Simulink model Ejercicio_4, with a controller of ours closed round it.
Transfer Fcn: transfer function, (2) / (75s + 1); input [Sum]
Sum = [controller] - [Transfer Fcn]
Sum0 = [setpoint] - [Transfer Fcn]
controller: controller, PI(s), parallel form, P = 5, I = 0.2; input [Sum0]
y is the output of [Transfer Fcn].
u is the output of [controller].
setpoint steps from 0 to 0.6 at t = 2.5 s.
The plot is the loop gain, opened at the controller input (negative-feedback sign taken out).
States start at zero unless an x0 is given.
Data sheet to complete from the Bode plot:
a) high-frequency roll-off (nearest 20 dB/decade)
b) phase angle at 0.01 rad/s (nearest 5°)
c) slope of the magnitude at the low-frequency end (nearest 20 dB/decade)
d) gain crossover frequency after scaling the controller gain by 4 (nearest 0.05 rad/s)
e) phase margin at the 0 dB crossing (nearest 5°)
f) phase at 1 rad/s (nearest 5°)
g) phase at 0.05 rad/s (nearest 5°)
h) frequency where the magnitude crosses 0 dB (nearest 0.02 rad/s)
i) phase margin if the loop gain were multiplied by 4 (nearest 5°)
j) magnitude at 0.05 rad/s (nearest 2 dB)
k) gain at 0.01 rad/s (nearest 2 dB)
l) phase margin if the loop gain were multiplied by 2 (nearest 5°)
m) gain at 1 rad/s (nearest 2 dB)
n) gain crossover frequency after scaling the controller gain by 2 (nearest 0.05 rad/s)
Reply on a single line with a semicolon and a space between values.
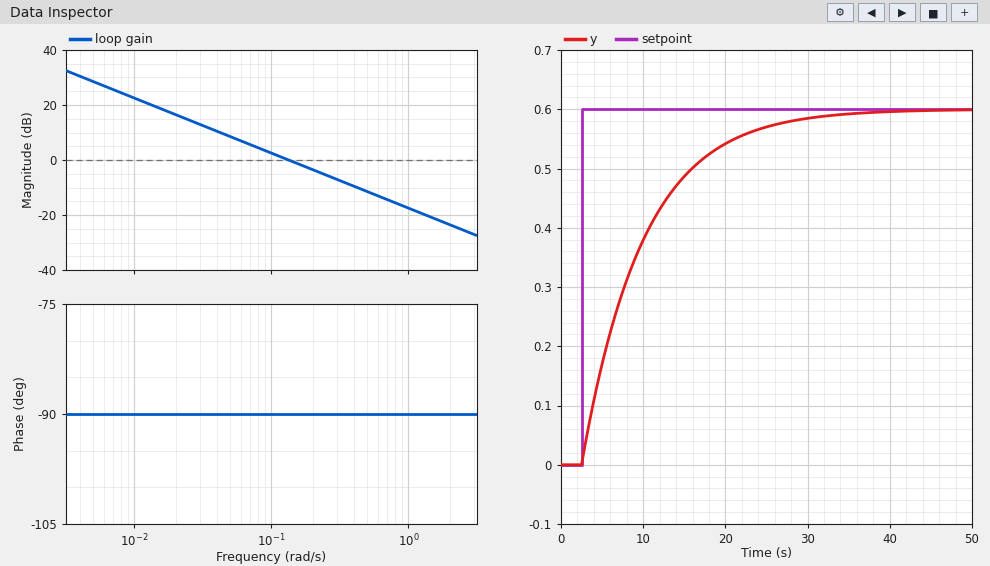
-20 dB/decade; -90°; -20 dB/decade; 0.55 rad/s; 90°; -90°; -90°; 0.14 rad/s; 90°; 8 dB; 22 dB; 90°; -18 dB; 0.25 rad/s
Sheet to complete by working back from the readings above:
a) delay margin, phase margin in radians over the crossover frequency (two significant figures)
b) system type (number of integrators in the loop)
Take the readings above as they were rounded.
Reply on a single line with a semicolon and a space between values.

11 s; 1
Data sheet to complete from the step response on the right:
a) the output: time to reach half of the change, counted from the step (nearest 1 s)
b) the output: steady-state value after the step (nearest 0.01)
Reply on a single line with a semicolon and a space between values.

5 s; 0.60
